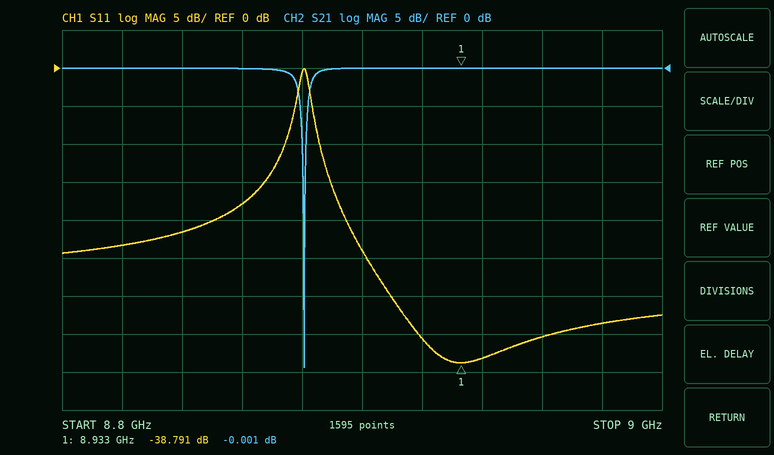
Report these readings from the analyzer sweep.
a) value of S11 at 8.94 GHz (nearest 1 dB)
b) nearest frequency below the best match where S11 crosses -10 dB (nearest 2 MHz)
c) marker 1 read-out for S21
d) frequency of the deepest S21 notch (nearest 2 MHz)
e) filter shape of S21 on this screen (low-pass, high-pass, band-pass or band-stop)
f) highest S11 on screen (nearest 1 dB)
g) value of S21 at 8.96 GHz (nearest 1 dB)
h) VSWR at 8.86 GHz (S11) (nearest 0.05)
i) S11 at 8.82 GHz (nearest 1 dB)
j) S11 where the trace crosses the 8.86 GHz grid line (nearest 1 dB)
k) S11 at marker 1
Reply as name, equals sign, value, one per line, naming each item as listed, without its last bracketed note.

value of S11 at 8.94 GHz = -38 dB
nearest frequency below the best match where S11 crosses -10 dB = 8.886 GHz
marker 1 read-out for S21 = -0.001 dB
frequency of the deepest S21 notch = 8.880 GHz
filter shape of S21 on this screen = band-stop
highest S11 on screen = 0 dB
value of S21 at 8.96 GHz = 0 dB
VSWR at 8.86 GHz (S11) = 1.30
S11 at 8.82 GHz = -23 dB
S11 where the trace crosses the 8.86 GHz grid line = -18 dB
S11 at marker 1 = -38.791 dB
